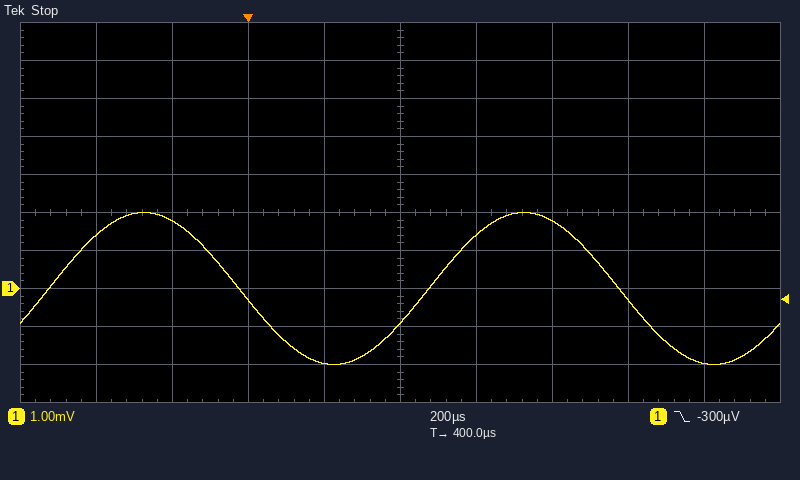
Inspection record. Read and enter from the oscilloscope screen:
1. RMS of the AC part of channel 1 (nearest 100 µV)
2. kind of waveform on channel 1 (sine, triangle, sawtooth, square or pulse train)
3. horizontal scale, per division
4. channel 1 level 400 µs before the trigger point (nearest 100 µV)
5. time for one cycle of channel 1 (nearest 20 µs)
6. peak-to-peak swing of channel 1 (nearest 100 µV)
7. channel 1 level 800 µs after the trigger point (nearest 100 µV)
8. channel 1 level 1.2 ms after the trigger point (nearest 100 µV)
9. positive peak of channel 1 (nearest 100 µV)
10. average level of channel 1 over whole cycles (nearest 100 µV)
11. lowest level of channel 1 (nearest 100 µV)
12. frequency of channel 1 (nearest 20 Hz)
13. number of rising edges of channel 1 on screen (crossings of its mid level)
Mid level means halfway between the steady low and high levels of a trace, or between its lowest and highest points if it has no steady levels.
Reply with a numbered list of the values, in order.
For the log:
1. 1.4 mV
2. sine
3. 200 µs
4. 1.4 mV
5. 1.00 ms
6. 4.0 mV
7. 1.8 mV
8. -2.0 mV
9. 2.0 mV
10. 0.0 mV
11. -2.0 mV
12. 1.00 kHz
13. 2
